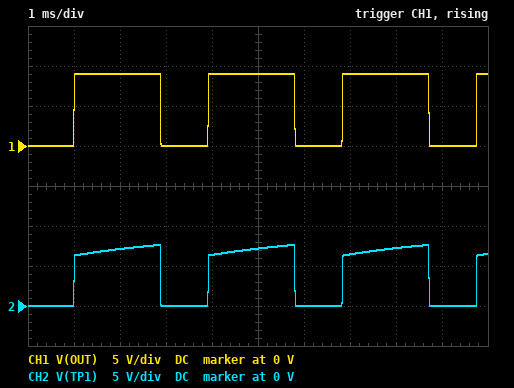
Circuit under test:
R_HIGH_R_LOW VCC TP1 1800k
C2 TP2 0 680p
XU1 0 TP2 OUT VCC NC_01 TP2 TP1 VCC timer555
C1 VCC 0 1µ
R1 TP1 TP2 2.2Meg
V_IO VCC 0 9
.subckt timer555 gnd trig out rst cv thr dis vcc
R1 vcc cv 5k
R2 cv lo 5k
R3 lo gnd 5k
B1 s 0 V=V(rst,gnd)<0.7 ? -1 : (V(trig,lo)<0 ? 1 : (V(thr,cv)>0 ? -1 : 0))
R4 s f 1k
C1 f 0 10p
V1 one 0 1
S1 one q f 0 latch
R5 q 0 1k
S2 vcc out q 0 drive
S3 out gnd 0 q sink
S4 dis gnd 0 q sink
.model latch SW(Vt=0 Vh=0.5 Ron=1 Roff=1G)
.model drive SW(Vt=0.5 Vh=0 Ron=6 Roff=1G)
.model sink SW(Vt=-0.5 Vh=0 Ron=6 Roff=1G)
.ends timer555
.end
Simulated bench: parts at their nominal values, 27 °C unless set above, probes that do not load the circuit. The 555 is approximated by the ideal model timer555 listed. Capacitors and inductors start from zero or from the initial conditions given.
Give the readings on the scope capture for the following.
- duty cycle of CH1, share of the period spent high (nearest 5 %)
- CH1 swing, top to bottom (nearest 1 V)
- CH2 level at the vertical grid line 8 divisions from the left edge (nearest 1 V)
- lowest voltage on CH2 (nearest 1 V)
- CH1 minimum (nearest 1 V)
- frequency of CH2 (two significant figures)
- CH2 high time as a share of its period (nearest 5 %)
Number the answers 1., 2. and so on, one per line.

1. 65 %
2. 9 V
3. 7 V
4. 0 V
5. 0 V
6. 340 Hz
7. 65 %
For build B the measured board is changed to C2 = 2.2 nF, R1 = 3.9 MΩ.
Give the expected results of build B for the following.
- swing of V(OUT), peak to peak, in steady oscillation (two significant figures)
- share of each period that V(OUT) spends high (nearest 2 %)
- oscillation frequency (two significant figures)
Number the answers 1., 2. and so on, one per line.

1. 9.0 V
2. 60 %
3. 68 Hz
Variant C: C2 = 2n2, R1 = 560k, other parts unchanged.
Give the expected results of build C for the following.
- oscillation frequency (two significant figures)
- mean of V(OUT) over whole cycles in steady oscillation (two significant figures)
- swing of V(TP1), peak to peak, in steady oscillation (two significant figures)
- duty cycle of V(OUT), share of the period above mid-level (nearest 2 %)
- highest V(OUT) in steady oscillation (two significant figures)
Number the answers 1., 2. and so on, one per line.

1. 220 Hz
2. 7.3 V
3. 6.7 V
4. 80 %
5. 9.0 V
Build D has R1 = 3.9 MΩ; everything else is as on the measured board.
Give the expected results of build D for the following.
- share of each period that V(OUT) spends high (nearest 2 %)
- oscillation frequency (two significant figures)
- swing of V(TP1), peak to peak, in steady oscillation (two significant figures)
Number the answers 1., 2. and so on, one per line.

1. 60 %
2. 220 Hz
3. 8.0 V
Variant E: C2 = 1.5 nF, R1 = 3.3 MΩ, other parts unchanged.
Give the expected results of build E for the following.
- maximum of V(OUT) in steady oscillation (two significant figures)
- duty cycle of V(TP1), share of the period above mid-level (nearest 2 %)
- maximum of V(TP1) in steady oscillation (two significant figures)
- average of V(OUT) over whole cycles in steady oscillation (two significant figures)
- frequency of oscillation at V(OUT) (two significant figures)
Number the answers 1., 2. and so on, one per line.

1. 9.0 V
2. 60 %
3. 7.9 V
4. 5.5 V
5. 110 Hz
